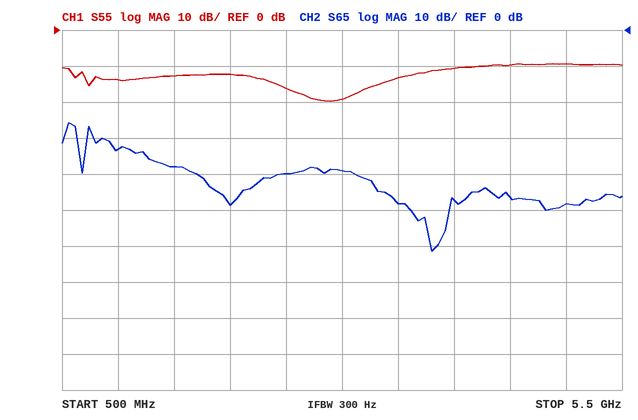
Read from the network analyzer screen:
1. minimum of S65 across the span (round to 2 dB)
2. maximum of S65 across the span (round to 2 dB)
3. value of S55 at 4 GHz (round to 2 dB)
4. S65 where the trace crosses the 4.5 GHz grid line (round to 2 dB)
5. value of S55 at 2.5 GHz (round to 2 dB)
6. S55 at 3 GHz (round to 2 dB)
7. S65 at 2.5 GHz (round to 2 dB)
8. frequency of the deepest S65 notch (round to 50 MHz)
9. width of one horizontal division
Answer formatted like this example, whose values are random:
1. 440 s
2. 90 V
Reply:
1. -62 dB
2. -26 dB
3. -10 dB
4. -46 dB
5. -16 dB
6. -20 dB
7. -40 dB
8. 3.80 GHz
9. 500 MHz
